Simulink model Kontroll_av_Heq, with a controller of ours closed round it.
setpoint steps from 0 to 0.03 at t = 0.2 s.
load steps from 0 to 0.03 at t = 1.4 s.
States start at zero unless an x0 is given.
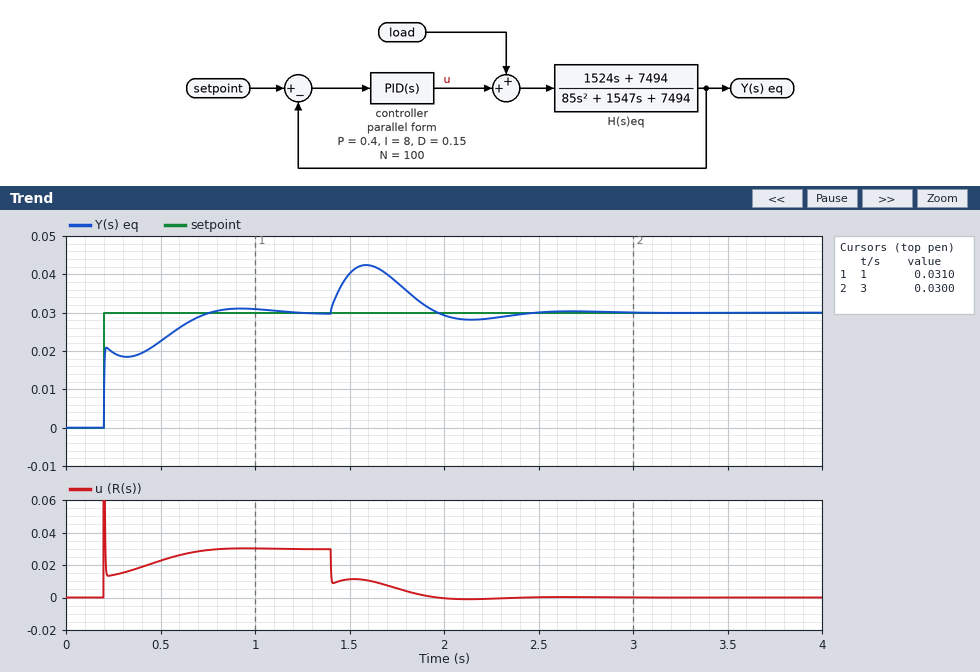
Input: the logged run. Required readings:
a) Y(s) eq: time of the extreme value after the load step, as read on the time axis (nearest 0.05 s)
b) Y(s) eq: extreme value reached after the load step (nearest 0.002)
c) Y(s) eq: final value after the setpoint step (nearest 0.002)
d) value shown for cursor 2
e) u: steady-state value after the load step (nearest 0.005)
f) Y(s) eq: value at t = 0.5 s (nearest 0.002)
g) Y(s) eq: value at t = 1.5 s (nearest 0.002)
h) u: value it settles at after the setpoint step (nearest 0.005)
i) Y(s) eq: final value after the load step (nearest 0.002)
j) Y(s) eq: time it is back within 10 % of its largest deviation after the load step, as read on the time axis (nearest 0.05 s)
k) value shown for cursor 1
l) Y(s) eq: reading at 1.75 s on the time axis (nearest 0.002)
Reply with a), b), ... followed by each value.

a) 1.60 s
b) 0.042
c) 0.030
d) 0.0300
e) 0.000
f) 0.022
g) 0.040
h) 0.030
i) 0.030
j) 2.30 s
k) 0.0310
l) 0.038
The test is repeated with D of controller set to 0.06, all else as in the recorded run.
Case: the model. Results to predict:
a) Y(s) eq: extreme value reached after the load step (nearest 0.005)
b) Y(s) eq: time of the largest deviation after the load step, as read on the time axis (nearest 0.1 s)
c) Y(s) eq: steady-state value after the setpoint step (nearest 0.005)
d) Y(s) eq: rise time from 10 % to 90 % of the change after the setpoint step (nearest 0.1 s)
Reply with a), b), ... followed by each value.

a) 0.045
b) 1.5 s
c) 0.030
d) 0.3 s
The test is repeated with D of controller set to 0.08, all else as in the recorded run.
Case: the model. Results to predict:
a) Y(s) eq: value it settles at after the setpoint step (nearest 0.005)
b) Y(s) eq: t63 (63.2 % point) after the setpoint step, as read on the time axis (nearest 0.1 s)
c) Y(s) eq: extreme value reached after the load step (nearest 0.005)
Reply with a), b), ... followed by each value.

a) 0.030
b) 0.4 s
c) 0.045
